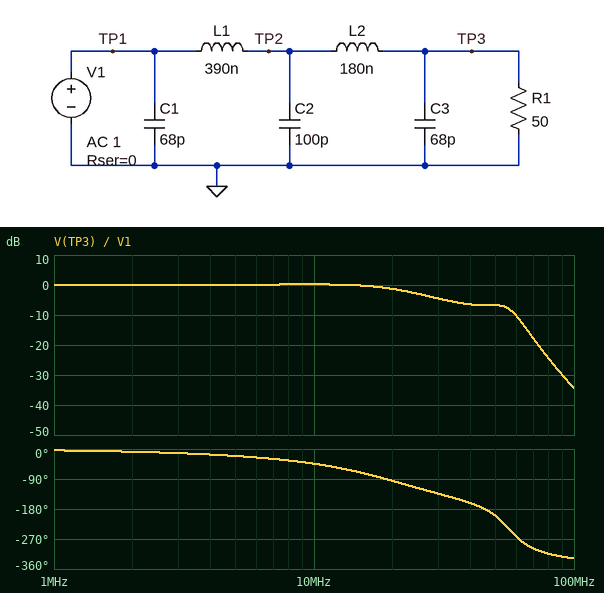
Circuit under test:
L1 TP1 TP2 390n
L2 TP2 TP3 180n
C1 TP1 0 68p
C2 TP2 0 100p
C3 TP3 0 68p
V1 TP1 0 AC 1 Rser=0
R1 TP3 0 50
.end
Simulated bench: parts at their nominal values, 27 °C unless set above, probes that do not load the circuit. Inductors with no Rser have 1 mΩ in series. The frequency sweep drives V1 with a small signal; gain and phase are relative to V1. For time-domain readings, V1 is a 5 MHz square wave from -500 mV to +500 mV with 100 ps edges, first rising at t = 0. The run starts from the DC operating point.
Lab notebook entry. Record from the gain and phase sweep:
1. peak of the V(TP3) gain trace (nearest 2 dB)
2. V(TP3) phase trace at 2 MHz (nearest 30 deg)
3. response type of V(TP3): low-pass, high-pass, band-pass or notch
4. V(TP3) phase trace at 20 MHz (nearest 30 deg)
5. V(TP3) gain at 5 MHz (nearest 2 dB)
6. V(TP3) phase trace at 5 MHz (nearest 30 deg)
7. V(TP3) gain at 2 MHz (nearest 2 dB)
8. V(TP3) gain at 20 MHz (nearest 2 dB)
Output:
0 dB
0 deg
low-pass
-90 deg
0 dB
-30 deg
0 dB
-2 dB
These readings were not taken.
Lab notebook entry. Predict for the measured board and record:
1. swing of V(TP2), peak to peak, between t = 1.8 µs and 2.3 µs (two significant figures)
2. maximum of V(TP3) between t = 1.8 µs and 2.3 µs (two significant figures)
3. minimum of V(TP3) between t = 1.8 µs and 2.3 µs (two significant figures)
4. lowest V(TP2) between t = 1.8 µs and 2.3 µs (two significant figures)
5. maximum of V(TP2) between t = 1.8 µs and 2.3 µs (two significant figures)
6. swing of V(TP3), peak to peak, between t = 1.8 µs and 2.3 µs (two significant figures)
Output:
1.2 V
580 mV
-580 mV
-580 mV
580 mV
1.2 V
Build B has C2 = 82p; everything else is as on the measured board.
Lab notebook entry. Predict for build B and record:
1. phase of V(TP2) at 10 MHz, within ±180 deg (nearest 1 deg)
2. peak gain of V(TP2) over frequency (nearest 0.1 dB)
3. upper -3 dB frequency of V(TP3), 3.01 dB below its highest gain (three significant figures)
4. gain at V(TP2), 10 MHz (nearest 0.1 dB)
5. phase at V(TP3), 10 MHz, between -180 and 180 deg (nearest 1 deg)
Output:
-30 deg
0 dB
24.4 MHz
-0.2 dB
-43 deg
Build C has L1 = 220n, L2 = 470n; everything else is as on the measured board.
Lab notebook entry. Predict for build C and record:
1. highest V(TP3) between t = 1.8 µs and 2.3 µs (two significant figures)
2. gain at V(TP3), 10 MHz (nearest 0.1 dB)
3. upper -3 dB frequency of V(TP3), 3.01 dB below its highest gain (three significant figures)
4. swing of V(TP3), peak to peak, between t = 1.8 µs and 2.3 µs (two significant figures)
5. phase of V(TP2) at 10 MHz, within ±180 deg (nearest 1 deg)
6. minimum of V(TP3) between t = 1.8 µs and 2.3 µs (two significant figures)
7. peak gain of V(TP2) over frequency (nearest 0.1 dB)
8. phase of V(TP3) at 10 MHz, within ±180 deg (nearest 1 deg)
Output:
620 mV
-0.8 dB
44.1 MHz
1.2 V
-14 deg
-620 mV
16.5 dB
-48 deg
